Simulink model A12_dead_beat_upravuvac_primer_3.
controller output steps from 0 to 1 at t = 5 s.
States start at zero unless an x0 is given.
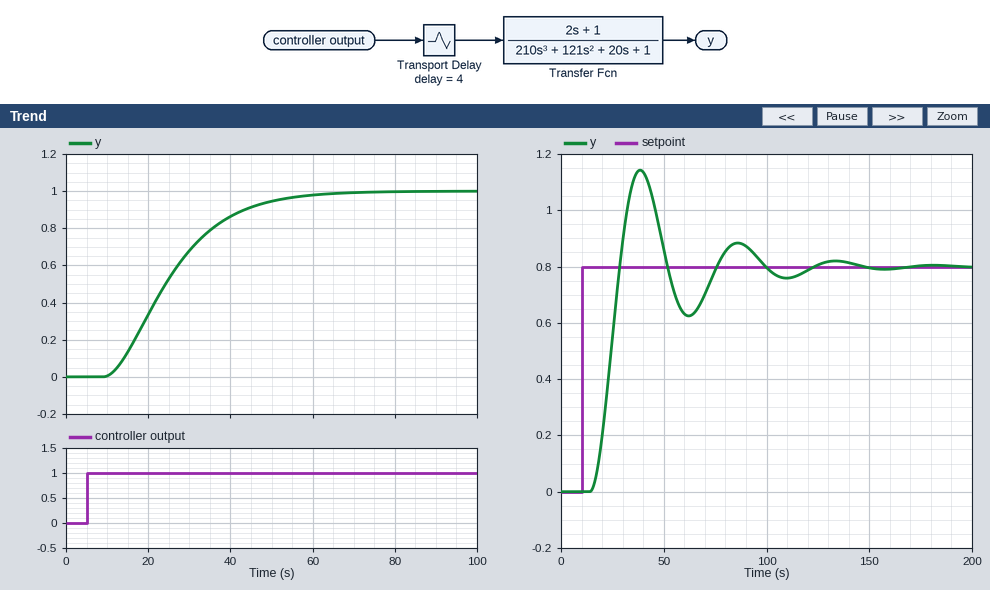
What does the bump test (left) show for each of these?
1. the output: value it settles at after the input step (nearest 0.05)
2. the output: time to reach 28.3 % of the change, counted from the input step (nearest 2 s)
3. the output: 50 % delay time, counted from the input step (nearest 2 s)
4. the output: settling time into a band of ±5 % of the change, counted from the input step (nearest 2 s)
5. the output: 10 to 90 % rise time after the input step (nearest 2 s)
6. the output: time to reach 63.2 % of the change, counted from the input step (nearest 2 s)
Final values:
1.00
14 s
20 s
46 s
30 s
24 s
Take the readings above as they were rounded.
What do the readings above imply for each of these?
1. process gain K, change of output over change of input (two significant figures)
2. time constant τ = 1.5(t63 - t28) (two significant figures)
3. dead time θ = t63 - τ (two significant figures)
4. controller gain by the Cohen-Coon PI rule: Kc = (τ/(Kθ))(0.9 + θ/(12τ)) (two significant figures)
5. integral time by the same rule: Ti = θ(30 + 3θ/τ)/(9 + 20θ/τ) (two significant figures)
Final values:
1.0
15 s
9.0 s
1.6
14 s
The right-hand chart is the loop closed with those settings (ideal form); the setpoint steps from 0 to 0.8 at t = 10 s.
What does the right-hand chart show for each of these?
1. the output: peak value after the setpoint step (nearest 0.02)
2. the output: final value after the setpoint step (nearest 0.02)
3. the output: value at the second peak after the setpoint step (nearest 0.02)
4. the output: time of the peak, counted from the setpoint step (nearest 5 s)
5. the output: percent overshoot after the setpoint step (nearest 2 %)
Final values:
1.14
0.80
0.88
30 s
42 %
